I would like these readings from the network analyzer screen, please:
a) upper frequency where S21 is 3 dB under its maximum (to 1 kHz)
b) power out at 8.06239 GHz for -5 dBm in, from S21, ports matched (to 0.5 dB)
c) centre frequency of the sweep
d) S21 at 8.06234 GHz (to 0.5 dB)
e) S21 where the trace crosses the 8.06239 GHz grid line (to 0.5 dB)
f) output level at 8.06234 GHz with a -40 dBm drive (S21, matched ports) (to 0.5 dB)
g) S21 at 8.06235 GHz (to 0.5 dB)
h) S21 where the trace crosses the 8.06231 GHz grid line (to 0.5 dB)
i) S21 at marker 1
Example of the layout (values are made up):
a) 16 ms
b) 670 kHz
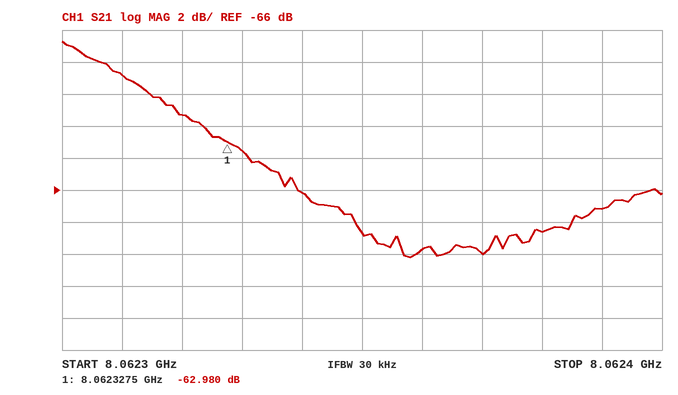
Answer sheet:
a) 8.062314 GHz
b) -72.0 dBm
c) 8.06235 GHz
d) -66.0 dB
e) -67.0 dB
f) -106.0 dBm
g) -68.5 dB
h) -59.0 dB
i) -62.980 dB
